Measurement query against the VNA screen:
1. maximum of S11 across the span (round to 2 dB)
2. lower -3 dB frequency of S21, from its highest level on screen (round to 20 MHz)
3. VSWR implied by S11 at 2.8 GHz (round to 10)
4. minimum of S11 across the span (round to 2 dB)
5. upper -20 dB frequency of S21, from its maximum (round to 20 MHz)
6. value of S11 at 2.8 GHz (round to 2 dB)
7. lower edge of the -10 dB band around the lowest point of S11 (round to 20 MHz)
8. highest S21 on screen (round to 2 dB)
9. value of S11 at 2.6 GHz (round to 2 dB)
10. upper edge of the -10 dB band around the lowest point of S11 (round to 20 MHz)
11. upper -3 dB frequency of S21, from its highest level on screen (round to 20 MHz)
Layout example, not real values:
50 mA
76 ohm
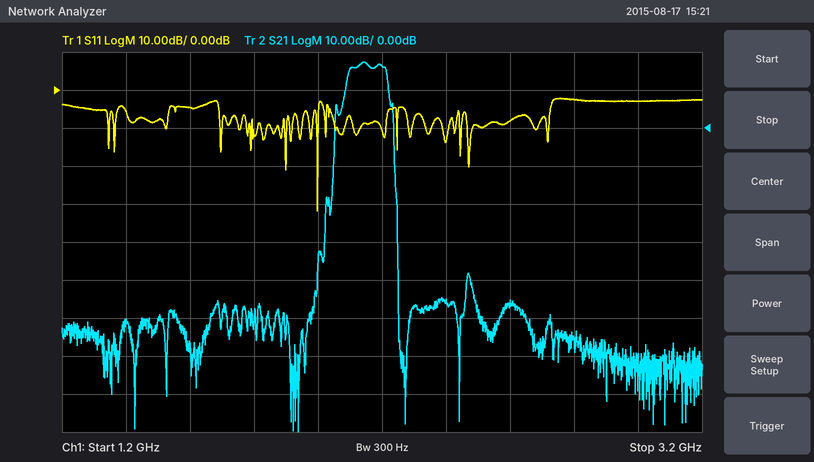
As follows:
-2 dB
2.10 GHz
10
-32 dB
2.24 GHz
-2 dB
2.00 GHz
18 dB
-8 dB
2.00 GHz
2.22 GHz
